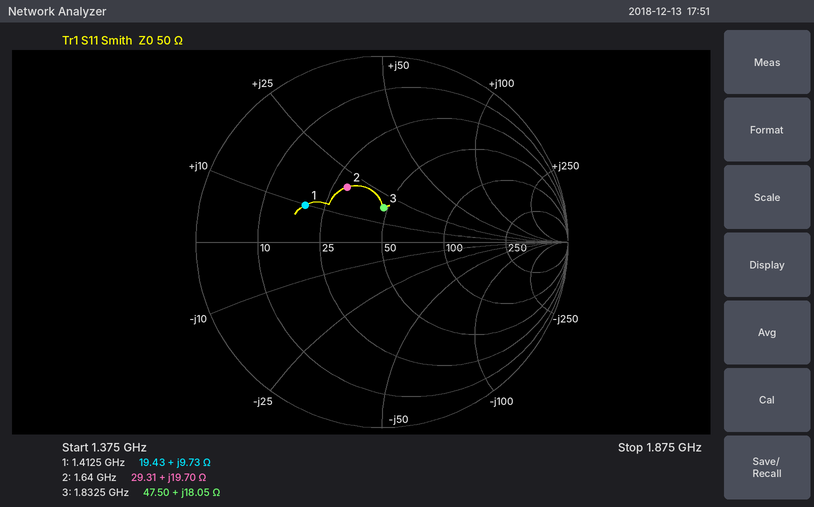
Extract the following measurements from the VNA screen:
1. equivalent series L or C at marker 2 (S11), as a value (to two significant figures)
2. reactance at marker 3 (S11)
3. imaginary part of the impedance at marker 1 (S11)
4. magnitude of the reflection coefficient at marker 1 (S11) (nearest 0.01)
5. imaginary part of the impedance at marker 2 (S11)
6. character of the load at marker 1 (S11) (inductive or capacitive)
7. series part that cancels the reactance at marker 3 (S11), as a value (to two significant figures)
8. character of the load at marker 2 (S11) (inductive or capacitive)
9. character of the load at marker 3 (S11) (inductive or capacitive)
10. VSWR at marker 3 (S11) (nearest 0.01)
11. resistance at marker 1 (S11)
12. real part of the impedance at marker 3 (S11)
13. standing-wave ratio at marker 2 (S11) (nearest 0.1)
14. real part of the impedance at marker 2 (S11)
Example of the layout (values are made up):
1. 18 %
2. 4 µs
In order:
1. 1.9 nH
2. +18.05 Ω
3. +9.73 Ω
4. 0.46
5. +19.70 Ω
6. inductive
7. 4.8 pF
8. inductive
9. inductive
10. 1.45
11. 19.43 Ω
12. 47.50 Ω
13. 2.1
14. 29.31 Ω
